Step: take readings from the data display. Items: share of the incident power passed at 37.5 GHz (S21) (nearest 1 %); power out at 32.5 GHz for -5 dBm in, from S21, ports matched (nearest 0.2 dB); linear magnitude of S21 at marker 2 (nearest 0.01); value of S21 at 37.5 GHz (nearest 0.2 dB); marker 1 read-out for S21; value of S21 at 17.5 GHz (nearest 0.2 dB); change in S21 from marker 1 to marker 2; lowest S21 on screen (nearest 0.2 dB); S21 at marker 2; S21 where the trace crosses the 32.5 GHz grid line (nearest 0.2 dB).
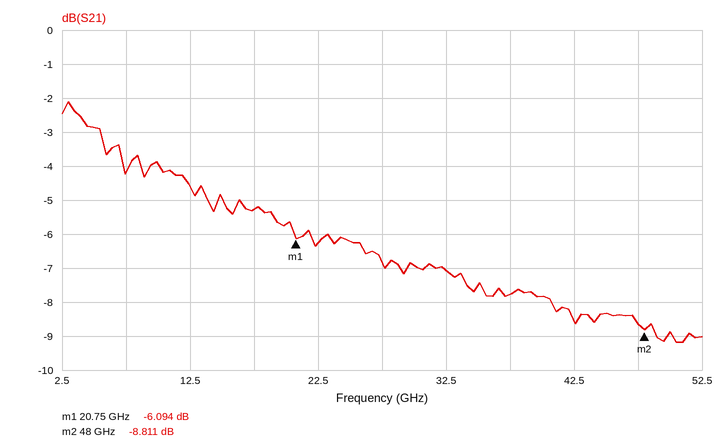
17 %
-12.0 dBm
0.36
-7.8 dB
-6.094 dB
-5.2 dB
-2.717 dB
-9.2 dB
-8.811 dB
-7.0 dB
